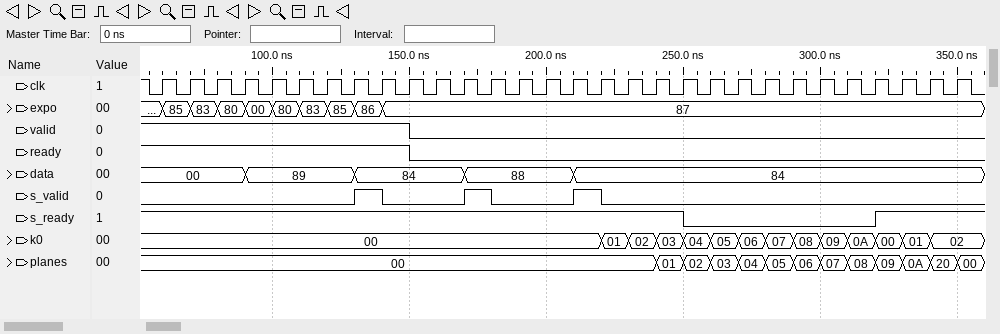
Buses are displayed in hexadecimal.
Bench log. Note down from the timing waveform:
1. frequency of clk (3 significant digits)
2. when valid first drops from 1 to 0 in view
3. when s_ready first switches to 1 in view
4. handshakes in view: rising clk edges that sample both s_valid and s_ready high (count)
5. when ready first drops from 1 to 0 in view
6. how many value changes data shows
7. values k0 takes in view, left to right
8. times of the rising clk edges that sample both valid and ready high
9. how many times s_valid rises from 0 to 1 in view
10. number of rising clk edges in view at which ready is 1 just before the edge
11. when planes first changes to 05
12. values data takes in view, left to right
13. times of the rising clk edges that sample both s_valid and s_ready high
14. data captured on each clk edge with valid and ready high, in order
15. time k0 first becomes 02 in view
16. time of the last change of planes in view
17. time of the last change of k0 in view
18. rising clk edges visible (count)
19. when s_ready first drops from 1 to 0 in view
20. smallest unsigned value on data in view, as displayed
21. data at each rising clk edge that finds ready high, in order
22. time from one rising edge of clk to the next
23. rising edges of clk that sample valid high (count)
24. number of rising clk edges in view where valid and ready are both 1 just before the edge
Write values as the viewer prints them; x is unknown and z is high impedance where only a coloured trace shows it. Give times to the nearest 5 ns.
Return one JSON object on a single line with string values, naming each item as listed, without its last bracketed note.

{"frequency of clk": "100 MHz", "when valid first drops from 1 to 0 in view": "150 ns", "when s_ready first switches to 1 in view": "320 ns", "handshakes in view: rising clk edges that sample both s_valid and s_ready high": "3", "when ready first drops from 1 to 0 in view": "150 ns", "how many value changes data shows": "4", "values k0 takes in view, left to right": "00, 01, 02, 03, 04, 05, 06, 07, 08, 09, 0A, 00, 01, 02", "times of the rising clk edges that sample both valid and ready high": "60 ns, 70 ns, 80 ns, 90 ns, 100 ns, 110 ns, 120 ns, 130 ns, 140 ns, 150 ns", "how many times s_valid rises from 0 to 1 in view": "3", "number of rising clk edges in view at which ready is 1 just before the edge": "10", "when planes first changes to 05": "280 ns", "values data takes in view, left to right": "00, 89, 84, 88, 84", "times of the rising clk edges that sample both s_valid and s_ready high": "140 ns, 180 ns, 220 ns", "data captured on each clk edge with valid and ready high, in order": "00, 00, 00, 00, 89, 89, 89, 89, 84, 84", "time k0 first becomes 02 in view": "230 ns", "time of the last change of planes in view": "350 ns", "time of the last change of k0 in view": "340 ns", "rising clk edges visible": "30", "when s_ready first drops from 1 to 0 in view": "250 ns", "smallest unsigned value on data in view, as displayed": "00", "data at each rising clk edge that finds ready high, in order": "00, 00, 00, 00, 89, 89, 89, 89, 84, 84", "time from one rising edge of clk to the next": "10 ns", "rising edges of clk that sample valid high": "10", "number of rising clk edges in view where valid and ready are both 1 just before the edge": "10"}
